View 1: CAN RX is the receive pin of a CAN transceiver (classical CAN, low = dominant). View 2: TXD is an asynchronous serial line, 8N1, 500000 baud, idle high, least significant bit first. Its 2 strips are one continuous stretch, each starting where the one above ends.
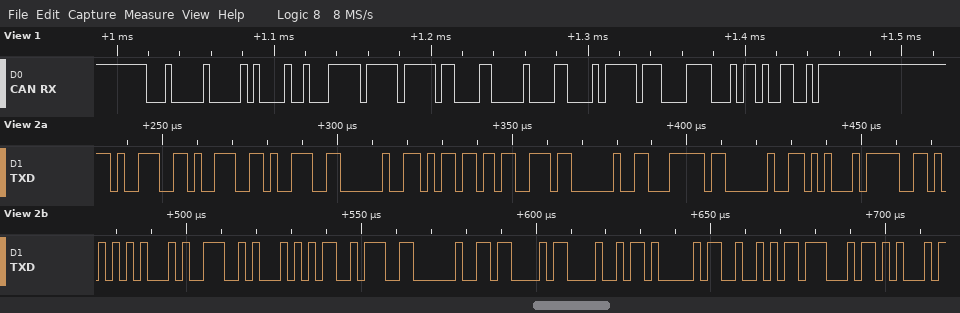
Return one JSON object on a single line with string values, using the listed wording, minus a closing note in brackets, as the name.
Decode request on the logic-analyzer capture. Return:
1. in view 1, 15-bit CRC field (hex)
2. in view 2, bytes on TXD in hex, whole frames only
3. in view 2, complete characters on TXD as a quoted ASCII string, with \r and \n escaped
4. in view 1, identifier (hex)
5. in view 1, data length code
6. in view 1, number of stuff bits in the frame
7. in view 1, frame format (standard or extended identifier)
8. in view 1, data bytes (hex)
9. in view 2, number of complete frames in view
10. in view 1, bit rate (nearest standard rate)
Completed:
{"in view 1, 15-bit CRC field": "0x0B4C", "in view 2, bytes on TXD in hex, whole frames only": "0x39 0x39 0x39 0x20 0x6D 0x73 0x20 0x7C 0x20 0x45 0x56 0x45 0x4E 0x54 0x3A 0x20 0x43 0x48 0x41 0x52 0x47 0x45", "in view 2, complete characters on TXD as a quoted ASCII string, with \\r and \\n escaped": "\"999 ms | EVENT: CHARGE\"", "in view 1, identifier": "0x100", "in view 1, data length code": "8", "in view 1, number of stuff bits in the frame": "7", "in view 1, frame format": "standard", "in view 1, data bytes": "48 FF FF 86 00 C2 FF 0F", "in view 2, number of complete frames in view": "22", "in view 1, bit rate": "250 kbit/s"}
